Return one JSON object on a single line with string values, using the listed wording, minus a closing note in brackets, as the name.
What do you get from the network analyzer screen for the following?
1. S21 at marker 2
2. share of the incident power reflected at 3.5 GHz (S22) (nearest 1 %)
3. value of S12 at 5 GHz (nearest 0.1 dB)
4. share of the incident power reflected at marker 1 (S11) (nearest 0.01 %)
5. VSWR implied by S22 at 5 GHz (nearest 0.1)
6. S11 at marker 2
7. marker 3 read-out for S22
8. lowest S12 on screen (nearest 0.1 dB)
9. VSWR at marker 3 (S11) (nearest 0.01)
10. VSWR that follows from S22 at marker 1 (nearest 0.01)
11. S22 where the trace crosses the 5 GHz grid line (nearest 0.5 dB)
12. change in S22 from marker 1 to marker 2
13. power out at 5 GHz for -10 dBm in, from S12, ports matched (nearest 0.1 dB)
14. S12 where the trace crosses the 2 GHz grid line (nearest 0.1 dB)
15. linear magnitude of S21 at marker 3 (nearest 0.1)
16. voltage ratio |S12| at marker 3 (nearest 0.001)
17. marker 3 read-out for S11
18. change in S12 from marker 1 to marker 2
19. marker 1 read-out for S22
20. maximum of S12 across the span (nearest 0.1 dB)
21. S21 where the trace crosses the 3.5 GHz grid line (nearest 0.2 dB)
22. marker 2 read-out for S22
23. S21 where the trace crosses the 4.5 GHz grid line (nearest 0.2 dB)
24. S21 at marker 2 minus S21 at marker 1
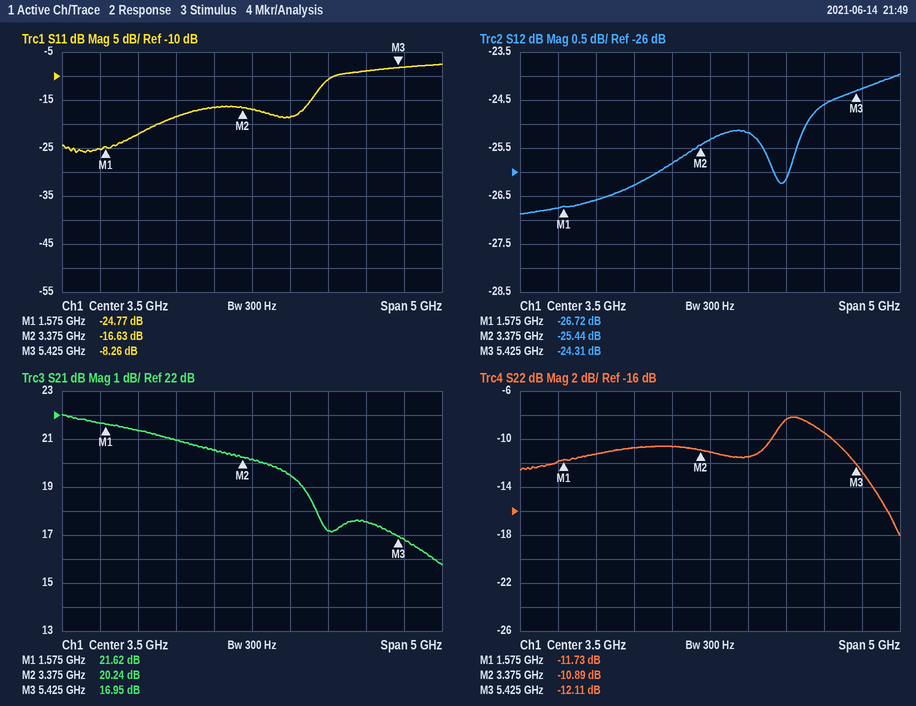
{"S21 at marker 2": "20.24 dB", "share of the incident power reflected at 3.5 GHz (S22)": "8 %", "value of S12 at 5 GHz": "-24.6 dB", "share of the incident power reflected at marker 1 (S11)": "0.33 %", "VSWR implied by S22 at 5 GHz": "2.0", "S11 at marker 2": "-16.63 dB", "marker 3 read-out for S22": "-12.11 dB", "lowest S12 on screen": "-26.9 dB", "VSWR at marker 3 (S11)": "2.26", "VSWR that follows from S22 at marker 1": "1.70", "S22 where the trace crosses the 5 GHz grid line": "-9.5 dB", "change in S22 from marker 1 to marker 2": "0.84 dB", "power out at 5 GHz for -10 dBm in, from S12, ports matched": "-34.6 dBm", "S12 where the trace crosses the 2 GHz grid line": "-26.6 dB", "linear magnitude of S21 at marker 3": "7.0", "voltage ratio |S12| at marker 3": "0.061", "marker 3 read-out for S11": "-8.26 dB", "change in S12 from marker 1 to marker 2": "1.28 dB", "marker 1 read-out for S22": "-11.73 dB", "maximum of S12 across the span": "-24.0 dB", "S21 where the trace crosses the 3.5 GHz grid line": "20.2 dB", "marker 2 read-out for S22": "-10.89 dB", "S21 where the trace crosses the 4.5 GHz grid line": "17.2 dB", "S21 at marker 2 minus S21 at marker 1": "-1.38 dB"}
